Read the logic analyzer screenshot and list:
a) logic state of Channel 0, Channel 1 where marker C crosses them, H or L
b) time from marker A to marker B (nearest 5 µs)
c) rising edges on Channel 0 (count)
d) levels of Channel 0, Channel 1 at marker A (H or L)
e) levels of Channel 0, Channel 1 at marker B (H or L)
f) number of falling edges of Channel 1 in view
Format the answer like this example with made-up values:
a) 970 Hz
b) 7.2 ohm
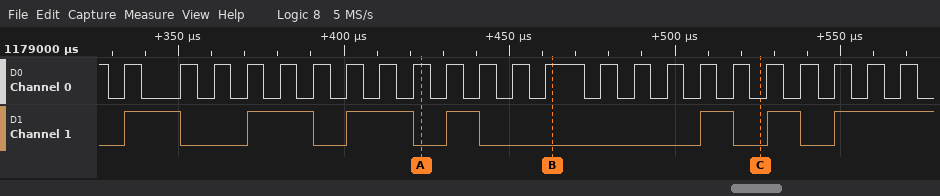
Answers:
a) Channel 0=L, Channel 1=L
b) 40 µs
c) 23
d) Channel 0=H, Channel 1=L
e) Channel 0=H, Channel 1=L
f) 6
